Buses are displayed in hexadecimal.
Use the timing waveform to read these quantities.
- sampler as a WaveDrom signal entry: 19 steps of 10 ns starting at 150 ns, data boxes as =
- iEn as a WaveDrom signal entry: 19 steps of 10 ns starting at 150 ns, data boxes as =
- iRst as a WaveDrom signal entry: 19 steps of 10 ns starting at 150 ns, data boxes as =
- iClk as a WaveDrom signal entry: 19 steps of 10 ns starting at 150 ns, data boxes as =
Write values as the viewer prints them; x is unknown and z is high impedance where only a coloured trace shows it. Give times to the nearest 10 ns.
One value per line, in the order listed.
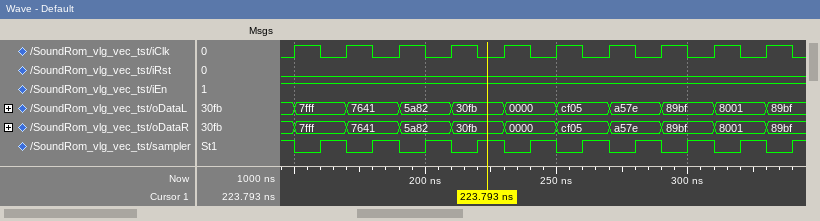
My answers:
{name: 'sampler', wave: '0101010101010101010'}
{name: 'iEn', wave: '1..................'}
{name: 'iRst', wave: '0..................'}
{name: 'iClk', wave: '1010101010101010101'}
